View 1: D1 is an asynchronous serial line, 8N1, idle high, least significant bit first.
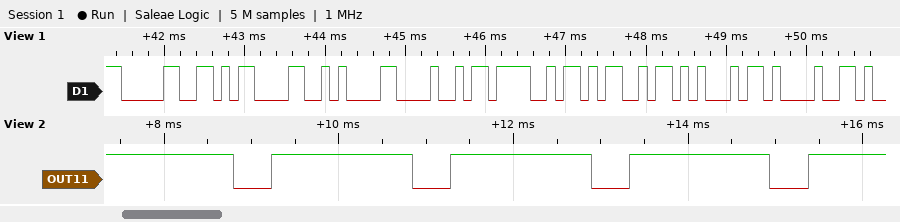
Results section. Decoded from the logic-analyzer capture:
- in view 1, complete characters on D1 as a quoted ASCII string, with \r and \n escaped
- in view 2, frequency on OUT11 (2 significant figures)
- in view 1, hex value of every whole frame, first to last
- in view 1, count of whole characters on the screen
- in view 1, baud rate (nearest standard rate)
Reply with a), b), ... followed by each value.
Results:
a) "0\r\nHOME!"
b) 490 Hz
c) 30 0D 0A 48 4F 4D 45 21
d) 8
e) 9600 baud
